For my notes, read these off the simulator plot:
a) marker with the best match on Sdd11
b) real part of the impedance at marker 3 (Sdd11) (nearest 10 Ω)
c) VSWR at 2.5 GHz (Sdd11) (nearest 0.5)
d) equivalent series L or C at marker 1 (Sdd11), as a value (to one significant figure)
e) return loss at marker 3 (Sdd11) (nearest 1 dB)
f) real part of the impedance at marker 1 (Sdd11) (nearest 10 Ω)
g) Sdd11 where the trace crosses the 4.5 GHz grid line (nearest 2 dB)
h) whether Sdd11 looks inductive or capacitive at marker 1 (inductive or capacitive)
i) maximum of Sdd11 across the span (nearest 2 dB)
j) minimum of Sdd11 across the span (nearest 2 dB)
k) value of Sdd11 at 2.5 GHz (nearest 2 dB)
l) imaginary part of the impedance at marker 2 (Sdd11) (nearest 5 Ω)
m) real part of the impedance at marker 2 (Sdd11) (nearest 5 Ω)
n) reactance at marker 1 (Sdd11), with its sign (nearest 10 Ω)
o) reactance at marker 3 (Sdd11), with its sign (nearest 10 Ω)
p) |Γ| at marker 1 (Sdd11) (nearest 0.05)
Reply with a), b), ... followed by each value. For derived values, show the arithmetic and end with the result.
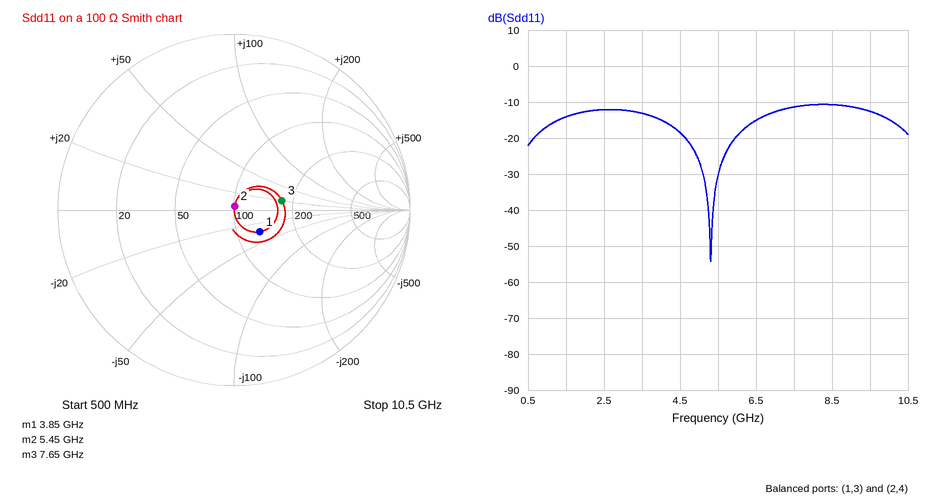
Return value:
a) marker 2
b) 170 Ω
c) |Γ| = 10^(-12/20) = 0.2512; VSWR = (1 + 0.2512)/(1 − 0.2512) ≈ 1.67, so 1.5 to the nearest 0.5
d) C = 1/(2π × 3.85 GHz × 30 Ω) ≈ 1 pF
e) 11 dB
f) 130 Ω
g) -18 dB
h) capacitive
i) -10 dB
j) -54 dB
k) -12 dB
l) +5 Ω
m) 100 Ω
n) -30 Ω
o) +20 Ω
p) 0.20
